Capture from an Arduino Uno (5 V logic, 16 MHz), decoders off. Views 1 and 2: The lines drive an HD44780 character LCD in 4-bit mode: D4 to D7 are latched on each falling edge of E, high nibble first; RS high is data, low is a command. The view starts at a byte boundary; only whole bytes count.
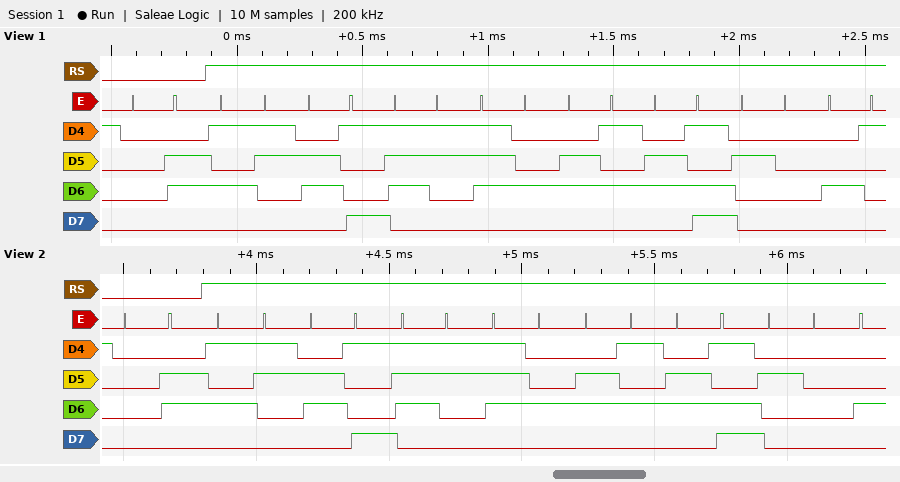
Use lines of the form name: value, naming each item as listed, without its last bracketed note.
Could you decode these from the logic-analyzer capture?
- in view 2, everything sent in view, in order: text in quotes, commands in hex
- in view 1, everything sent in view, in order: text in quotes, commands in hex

in view 2, everything sent in view, in order: text in quotes, commands in hex: 0x06 "Sistem "
in view 1, everything sent in view, in order: text in quotes, commands in hex: 0x06 "Sistem A"
